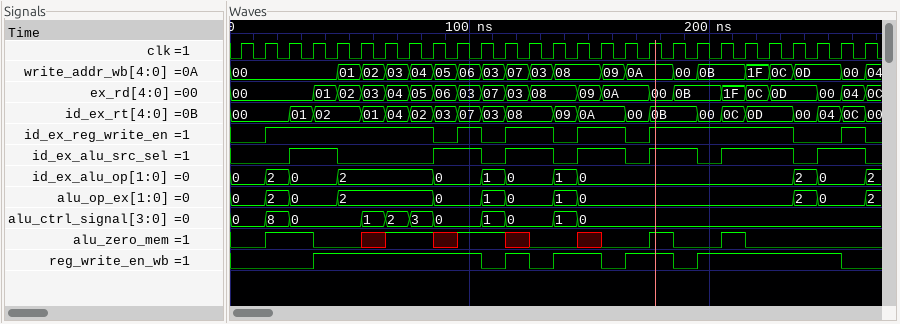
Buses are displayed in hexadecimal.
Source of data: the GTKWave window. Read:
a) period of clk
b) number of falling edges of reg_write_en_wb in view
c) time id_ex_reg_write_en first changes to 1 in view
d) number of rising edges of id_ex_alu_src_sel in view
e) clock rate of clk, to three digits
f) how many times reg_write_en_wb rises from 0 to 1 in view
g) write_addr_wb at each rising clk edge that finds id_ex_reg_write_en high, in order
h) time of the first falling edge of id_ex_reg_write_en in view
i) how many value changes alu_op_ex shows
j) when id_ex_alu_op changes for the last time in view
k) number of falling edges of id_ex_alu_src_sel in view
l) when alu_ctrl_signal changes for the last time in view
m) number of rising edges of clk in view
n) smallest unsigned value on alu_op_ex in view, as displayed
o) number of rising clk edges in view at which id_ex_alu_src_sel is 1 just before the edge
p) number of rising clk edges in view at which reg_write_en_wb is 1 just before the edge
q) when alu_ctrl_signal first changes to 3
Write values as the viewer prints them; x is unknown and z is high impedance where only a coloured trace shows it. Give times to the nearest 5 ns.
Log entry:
10 ns
5
15 ns
7
100 MHz
5
00, 00, 00, 01, 02, 03, 04, 06, 07, 03, 08, 09, 0A, 00, 0B, 0B, 1F, 0C, 00
85 ns
11
265 ns
7
145 ns
27
0
15
18
75 ns
